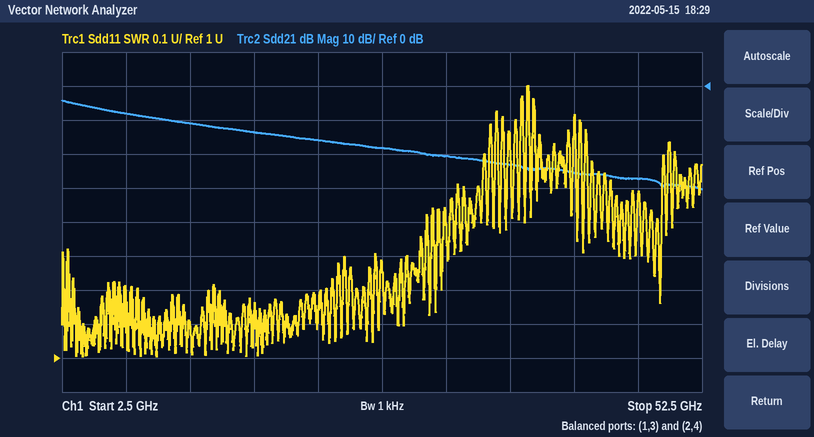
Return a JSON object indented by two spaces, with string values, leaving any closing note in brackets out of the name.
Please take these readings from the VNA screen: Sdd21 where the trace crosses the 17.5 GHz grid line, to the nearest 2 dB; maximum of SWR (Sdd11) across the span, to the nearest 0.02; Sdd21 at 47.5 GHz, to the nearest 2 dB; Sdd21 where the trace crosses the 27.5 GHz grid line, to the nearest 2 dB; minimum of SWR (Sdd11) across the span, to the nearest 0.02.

{
  "Sdd21 where the trace crosses the 17.5 GHz grid line, to the nearest 2 dB": "-14 dB",
  "maximum of SWR (Sdd11) across the span, to the nearest 0.02": "1.80",
  "Sdd21 at 47.5 GHz, to the nearest 2 dB": "-28 dB",
  "Sdd21 where the trace crosses the 27.5 GHz grid line, to the nearest 2 dB": "-18 dB",
  "minimum of SWR (Sdd11) across the span, to the nearest 0.02": "1.00"
}
